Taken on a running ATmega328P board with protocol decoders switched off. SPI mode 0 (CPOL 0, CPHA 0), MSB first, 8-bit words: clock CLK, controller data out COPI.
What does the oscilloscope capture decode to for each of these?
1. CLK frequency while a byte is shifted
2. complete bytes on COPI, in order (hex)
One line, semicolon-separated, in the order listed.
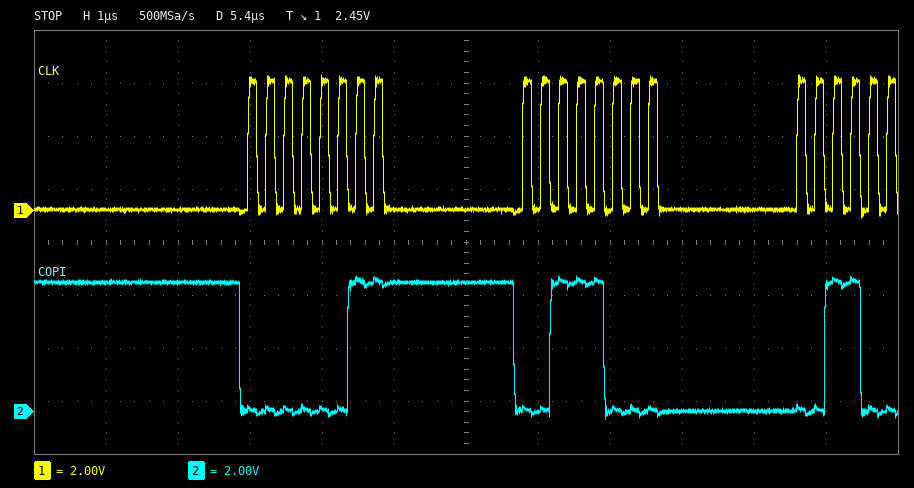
4 MHz; 03 38
